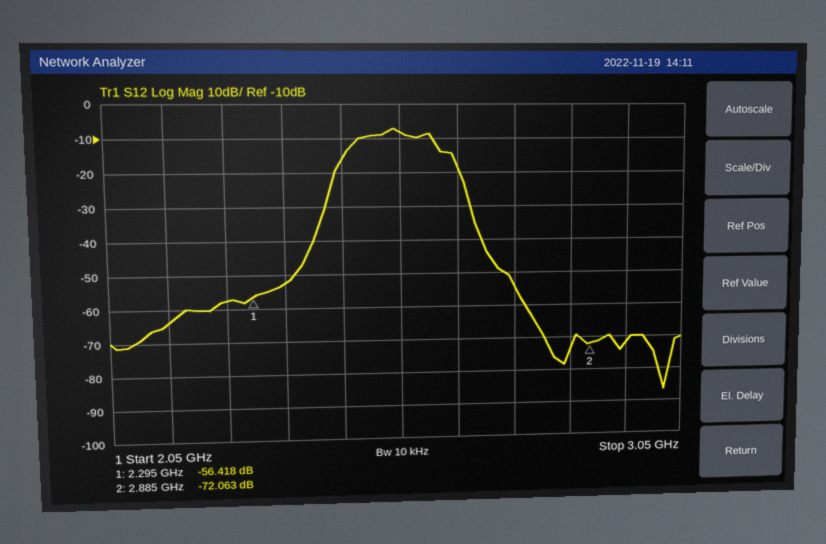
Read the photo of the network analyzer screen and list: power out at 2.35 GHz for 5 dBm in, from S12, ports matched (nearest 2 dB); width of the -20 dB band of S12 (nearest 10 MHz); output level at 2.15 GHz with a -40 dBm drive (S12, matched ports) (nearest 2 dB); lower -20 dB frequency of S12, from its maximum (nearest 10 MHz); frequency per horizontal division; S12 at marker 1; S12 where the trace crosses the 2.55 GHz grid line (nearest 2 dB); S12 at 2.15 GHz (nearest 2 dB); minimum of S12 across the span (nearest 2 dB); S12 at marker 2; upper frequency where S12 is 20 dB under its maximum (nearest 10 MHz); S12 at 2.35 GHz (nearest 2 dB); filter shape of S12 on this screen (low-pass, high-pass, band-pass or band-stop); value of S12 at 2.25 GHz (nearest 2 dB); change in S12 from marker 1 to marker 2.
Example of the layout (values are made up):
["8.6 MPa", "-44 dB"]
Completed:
["-48 dBm", "240 MHz", "-104 dBm", "2.43 GHz", "100 MHz", "-56.418 dB", "-8 dB", "-64 dB", "-86 dB", "-72.063 dB", "2.67 GHz", "-52 dB", "band-pass", "-58 dB", "-15.645 dB"]
